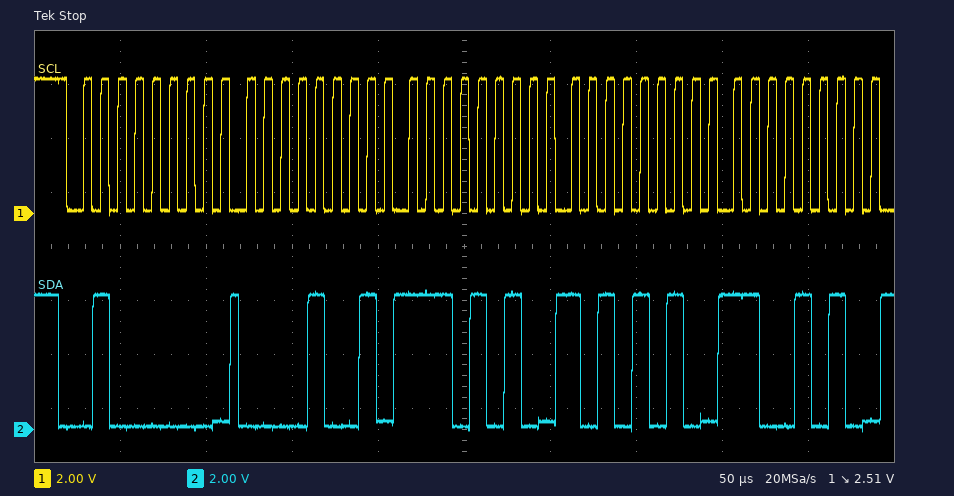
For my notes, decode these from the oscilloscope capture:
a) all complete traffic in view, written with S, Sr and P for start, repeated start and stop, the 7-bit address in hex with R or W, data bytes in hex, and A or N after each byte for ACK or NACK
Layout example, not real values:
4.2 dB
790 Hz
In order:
S 20W A 09 A EA A AA A CA A
